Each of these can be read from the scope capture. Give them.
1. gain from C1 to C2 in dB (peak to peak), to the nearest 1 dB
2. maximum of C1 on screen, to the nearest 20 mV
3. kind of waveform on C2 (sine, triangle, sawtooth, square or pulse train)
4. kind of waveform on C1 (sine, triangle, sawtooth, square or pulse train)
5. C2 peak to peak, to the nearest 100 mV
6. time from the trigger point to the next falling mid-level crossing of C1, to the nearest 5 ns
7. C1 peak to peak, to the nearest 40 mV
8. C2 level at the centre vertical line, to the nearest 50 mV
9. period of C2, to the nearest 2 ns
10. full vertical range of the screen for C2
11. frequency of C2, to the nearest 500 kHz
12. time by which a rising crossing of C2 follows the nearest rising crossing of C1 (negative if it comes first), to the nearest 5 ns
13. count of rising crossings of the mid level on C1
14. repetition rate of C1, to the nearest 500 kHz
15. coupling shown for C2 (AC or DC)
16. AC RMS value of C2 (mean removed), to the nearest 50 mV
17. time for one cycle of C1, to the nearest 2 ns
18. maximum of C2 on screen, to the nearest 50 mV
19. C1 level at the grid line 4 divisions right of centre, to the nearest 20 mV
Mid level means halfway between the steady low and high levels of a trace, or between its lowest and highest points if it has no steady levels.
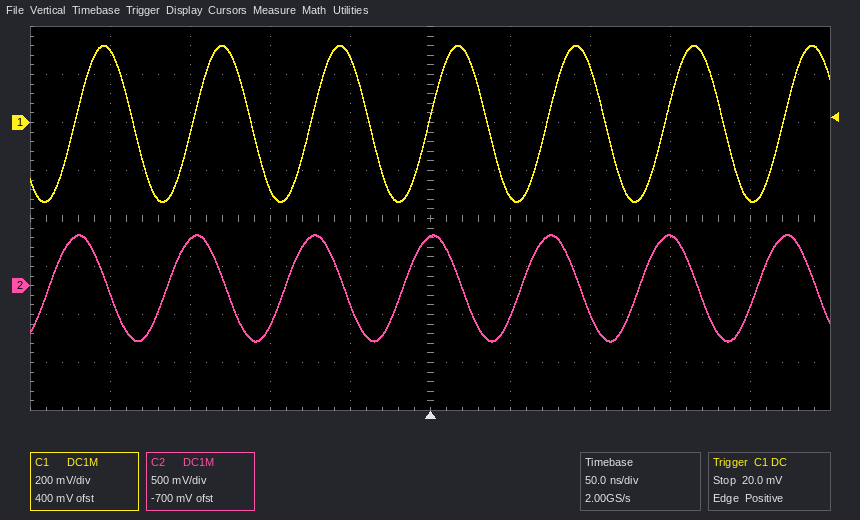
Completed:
5 dB
320 mV
sine
sine
1.10 V
35 ns
640 mV
500 mV
74 ns
4 V
13.5 MHz
-15 ns
7
13.5 MHz
DC
400 mV
74 ns
550 mV
-320 mV
